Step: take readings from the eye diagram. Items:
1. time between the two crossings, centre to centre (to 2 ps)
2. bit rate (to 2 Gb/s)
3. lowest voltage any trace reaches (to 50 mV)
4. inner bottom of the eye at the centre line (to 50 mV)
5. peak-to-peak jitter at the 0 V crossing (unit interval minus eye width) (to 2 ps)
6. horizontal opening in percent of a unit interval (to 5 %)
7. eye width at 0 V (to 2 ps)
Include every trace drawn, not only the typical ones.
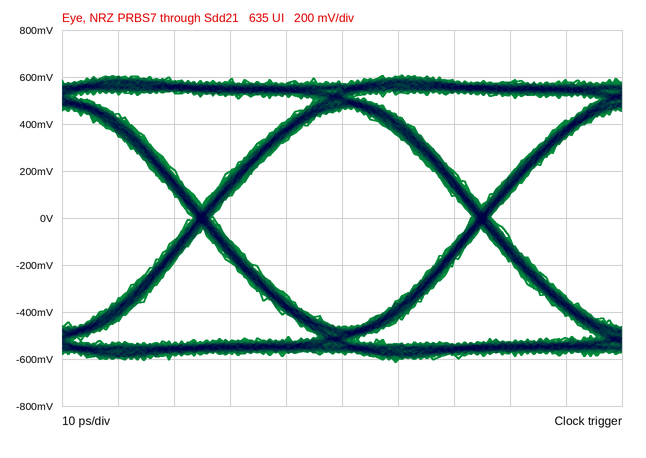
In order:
50 ps
20 Gb/s
-600 mV
-450 mV
4 ps
90 %
46 ps
